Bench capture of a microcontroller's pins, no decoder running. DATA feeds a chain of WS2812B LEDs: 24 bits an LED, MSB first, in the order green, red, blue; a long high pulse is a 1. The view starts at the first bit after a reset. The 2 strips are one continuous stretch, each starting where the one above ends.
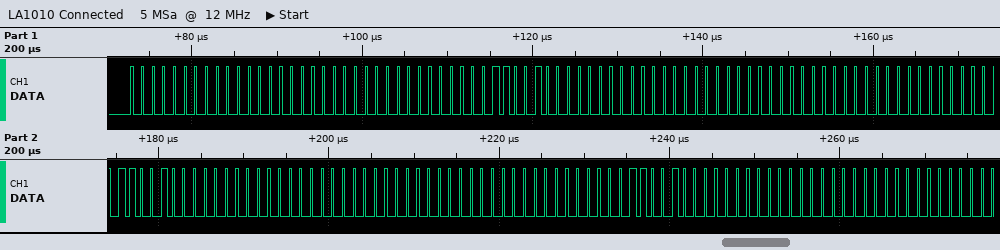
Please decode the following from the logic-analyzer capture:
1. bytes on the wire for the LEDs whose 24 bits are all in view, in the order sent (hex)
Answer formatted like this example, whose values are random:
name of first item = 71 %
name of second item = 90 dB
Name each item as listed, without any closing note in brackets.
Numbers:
bytes on the wire for the LEDs whose 24 bits are all in view, in the order sent = 00 00 00 00 32 00 00 00 00 00 32 00 00 00 00 00 32 00
